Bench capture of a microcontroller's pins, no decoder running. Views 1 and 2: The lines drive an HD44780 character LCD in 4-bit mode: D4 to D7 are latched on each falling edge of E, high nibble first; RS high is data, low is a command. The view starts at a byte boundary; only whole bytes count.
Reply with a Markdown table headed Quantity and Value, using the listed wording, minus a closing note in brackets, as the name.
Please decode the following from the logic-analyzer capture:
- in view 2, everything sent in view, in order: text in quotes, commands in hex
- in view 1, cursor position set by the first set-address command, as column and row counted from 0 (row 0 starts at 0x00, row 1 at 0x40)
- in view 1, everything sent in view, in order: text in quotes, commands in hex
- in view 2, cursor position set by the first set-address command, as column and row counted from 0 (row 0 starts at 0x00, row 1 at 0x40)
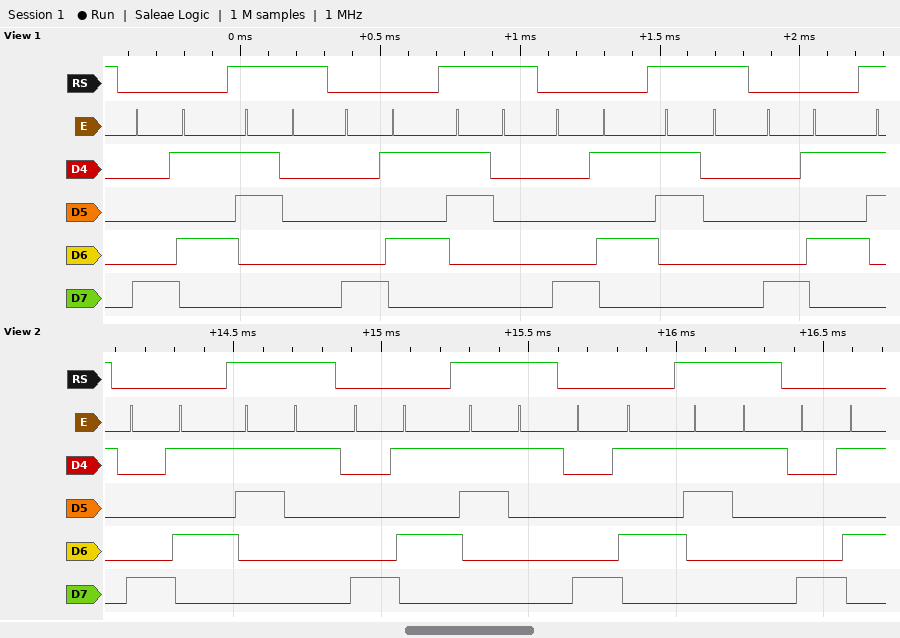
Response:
| Quantity | Value |
|---|---|
| in view 2, everything sent in view, in order: text in quotes, commands in hex | 0x85 "1" 0x85 "1" 0x85 "1" 0x85 |
| in view 1, cursor position set by the first set-address command, as column and row counted from 0 | column 5, row 0 |
| in view 1, everything sent in view, in order: text in quotes, commands in hex | 0x85 "0" 0x85 "0" 0x85 "0" 0x85 |
| in view 2, cursor position set by the first set-address command, as column and row counted from 0 | column 5, row 0 |
